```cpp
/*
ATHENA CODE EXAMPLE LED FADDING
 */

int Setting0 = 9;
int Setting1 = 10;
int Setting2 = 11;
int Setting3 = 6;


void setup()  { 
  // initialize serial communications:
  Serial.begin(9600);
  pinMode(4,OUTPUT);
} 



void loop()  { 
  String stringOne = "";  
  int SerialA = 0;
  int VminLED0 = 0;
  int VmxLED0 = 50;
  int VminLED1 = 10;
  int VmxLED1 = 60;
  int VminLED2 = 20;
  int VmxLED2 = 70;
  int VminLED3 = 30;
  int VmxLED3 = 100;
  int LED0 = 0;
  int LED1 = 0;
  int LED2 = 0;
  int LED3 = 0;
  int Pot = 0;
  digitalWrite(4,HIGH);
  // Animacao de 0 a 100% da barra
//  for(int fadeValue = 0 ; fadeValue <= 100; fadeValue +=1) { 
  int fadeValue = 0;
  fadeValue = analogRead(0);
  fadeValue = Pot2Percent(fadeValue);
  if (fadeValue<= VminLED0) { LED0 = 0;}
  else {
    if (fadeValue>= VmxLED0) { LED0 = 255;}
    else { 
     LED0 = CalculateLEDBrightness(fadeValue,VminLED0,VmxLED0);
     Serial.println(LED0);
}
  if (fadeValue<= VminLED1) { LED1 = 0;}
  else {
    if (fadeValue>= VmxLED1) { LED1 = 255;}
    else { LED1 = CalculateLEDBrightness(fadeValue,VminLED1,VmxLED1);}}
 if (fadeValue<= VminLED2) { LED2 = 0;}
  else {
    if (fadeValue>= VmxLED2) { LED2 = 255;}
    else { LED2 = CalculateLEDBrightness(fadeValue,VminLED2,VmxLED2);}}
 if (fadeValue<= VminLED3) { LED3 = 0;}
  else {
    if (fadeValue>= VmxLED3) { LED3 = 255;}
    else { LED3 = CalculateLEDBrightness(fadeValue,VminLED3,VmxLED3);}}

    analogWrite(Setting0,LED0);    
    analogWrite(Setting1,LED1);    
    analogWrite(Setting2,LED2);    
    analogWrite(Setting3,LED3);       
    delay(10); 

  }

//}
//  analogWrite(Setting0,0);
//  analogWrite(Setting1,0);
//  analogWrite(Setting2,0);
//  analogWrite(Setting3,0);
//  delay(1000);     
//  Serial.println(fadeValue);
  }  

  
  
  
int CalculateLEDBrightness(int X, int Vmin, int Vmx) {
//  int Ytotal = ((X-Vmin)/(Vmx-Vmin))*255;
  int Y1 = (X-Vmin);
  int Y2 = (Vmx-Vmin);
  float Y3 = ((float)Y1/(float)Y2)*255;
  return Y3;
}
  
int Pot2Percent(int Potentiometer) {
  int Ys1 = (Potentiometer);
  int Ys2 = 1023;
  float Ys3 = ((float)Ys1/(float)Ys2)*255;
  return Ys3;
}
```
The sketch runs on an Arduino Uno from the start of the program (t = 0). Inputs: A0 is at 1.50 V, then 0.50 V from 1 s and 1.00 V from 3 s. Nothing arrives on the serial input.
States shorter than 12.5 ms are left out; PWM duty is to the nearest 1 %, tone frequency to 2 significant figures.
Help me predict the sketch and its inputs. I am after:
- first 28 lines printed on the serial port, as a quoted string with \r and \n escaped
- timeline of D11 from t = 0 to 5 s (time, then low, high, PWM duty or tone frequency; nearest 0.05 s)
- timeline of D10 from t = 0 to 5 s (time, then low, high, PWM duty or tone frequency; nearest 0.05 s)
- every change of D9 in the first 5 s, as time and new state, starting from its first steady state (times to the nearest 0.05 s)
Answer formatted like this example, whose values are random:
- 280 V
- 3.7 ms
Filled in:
- "127\r\n127\r\n127\r\n127\r\n127\r\n127\r\n127\r\n127\r\n127\r\n127\r\n127\r\n127\r\n127\r\n127\r\n127\r\n127\r\n127\r\n127\r\n127\r\n127\r\n127\r\n127\r\n127\r\n127\r\n127\r\n127\r\n127\r\n127\r\n"
- 0 s high; 1 s PWM 10 %; 3 s PWM 60 %
- 0 s high; 1 s PWM 30 %; 3 s PWM 80 %
- 0 s high; 1 s PWM 50 %; 3 s high
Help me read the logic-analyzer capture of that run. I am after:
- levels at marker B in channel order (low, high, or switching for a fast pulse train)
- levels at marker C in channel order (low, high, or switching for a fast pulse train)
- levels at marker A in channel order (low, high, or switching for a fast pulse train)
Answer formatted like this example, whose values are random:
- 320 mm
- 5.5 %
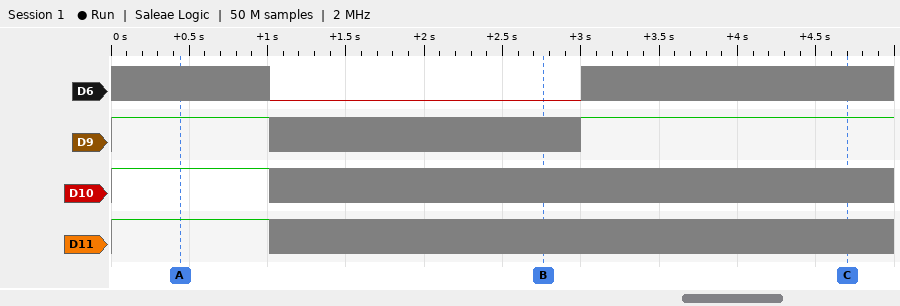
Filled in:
- D6 low, D9 switching, D10 switching, D11 switching
- D6 switching, D9 high, D10 switching, D11 switching
- D6 switching, D9 high, D10 high, D11 high
